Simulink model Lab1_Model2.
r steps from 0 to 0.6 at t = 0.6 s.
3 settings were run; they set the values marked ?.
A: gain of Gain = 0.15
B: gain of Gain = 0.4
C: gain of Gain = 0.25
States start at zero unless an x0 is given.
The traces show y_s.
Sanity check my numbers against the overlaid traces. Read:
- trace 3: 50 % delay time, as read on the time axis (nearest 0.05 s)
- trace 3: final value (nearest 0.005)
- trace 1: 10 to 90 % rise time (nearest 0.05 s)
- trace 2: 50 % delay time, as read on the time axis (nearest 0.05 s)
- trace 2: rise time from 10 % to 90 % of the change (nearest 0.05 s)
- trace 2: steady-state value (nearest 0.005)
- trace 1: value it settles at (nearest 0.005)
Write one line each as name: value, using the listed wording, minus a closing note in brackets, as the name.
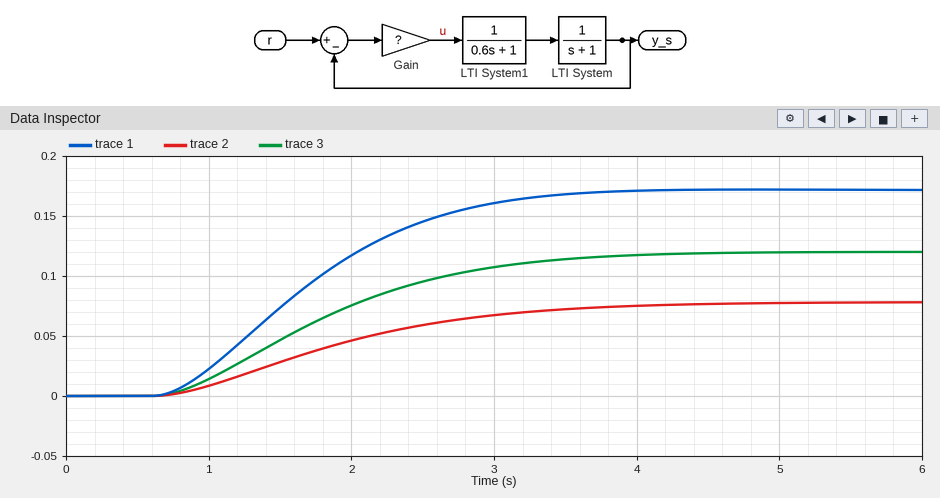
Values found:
trace 3: 50 % delay time, as read on the time axis: 1.70 s
trace 3: final value: 0.120
trace 1: 10 to 90 % rise time: 1.80 s
trace 2: 50 % delay time, as read on the time axis: 1.80 s
trace 2: rise time from 10 % to 90 % of the change: 2.30 s
trace 2: steady-state value: 0.080
trace 1: value it settles at: 0.170
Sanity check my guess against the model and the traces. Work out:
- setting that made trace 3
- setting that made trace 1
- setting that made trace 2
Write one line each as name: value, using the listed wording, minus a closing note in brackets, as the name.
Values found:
setting that made trace 3: C
setting that made trace 1: B
setting that made trace 2: A
